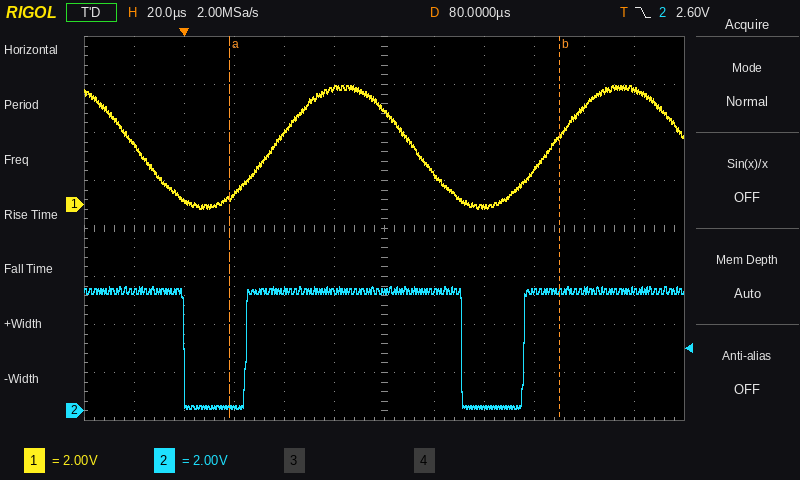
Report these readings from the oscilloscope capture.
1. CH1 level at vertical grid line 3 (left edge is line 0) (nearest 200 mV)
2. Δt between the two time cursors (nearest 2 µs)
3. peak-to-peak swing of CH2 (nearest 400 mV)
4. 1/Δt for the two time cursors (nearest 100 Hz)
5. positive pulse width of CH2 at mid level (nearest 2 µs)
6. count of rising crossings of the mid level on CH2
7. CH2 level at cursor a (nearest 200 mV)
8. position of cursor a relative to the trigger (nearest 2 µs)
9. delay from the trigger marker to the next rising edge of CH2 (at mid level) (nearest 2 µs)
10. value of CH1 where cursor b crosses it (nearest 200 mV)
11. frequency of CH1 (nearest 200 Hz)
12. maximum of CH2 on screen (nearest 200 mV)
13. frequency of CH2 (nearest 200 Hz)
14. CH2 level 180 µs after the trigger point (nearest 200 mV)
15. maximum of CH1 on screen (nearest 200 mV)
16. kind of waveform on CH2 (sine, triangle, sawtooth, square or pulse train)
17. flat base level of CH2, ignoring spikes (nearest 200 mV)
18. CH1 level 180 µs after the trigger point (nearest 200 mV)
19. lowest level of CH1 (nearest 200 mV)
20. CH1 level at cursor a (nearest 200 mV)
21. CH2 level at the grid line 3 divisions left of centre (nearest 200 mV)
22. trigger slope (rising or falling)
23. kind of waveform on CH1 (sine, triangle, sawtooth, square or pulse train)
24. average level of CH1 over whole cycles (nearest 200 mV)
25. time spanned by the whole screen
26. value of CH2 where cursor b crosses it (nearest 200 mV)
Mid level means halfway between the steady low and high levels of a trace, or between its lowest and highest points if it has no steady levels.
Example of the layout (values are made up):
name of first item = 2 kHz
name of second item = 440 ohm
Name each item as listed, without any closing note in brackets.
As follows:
CH1 level at vertical grid line 3 (left edge is line 0) = 400 mV
Δt between the two time cursors = 132 µs
peak-to-peak swing of CH2 = 5.2 V
1/Δt for the two time cursors = 7.6 kHz
positive pulse width of CH2 at mid level = 86 µs
count of rising crossings of the mid level on CH2 = 2
CH2 level at cursor a = 200 mV
position of cursor a relative to the trigger = +18 µs
delay from the trigger marker to the next rising edge of CH2 (at mid level) = 24 µs
value of CH1 where cursor b crosses it = 2.8 V
frequency of CH1 = 9.0 kHz
maximum of CH2 on screen = 5.2 V
frequency of CH2 = 9.0 kHz
CH2 level 180 µs after the trigger point = 5.0 V
maximum of CH1 on screen = 5.0 V
kind of waveform on CH2 = pulse train
flat base level of CH2, ignoring spikes = 200 mV
CH1 level 180 µs after the trigger point = 4.8 V
lowest level of CH1 = -200 mV
CH1 level at cursor a = 200 mV
CH2 level at the grid line 3 divisions left of centre = 200 mV
trigger slope = falling
kind of waveform on CH1 = sine
average level of CH1 over whole cycles = 2.4 V
time spanned by the whole screen = 240 µs
value of CH2 where cursor b crosses it = 5.0 V
